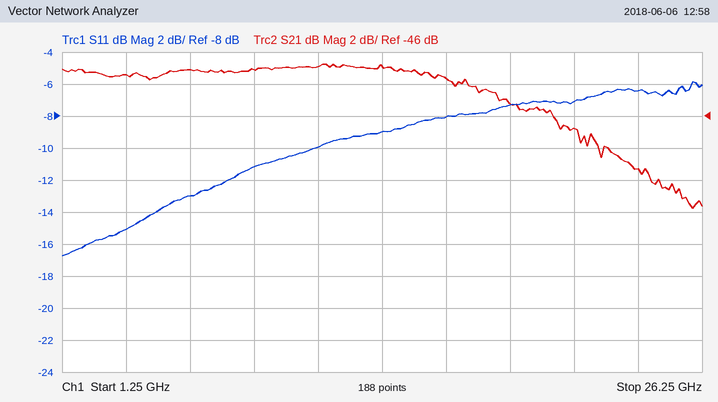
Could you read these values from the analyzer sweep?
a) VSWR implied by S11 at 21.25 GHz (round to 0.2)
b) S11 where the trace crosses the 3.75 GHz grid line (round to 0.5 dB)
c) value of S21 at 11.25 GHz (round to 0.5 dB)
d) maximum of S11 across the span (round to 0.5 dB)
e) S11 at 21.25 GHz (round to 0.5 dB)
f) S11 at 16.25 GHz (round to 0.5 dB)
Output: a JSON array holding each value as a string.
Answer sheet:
["2.6", "-15.0 dB", "-43.0 dB", "-6.0 dB", "-7.0 dB", "-8.0 dB"]
